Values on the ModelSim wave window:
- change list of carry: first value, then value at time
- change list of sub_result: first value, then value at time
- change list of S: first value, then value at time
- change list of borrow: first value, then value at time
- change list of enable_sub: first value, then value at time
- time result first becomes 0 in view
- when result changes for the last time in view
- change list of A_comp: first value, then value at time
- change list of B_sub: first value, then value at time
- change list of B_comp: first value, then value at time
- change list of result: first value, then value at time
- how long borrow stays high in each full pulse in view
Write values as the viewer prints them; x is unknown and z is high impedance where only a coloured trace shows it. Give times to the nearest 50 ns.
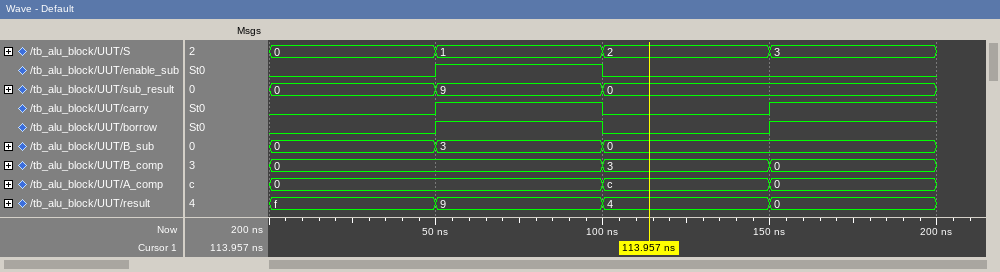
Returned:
0, 1 at 50 ns, 0 at 100 ns, 1 at 150 ns
0, 9 at 50 ns, 0 at 100 ns
0, 1 at 50 ns, 2 at 100 ns, 3 at 150 ns
0, 1 at 50 ns, 0 at 100 ns, 1 at 150 ns
0, 1 at 50 ns, 0 at 100 ns
150 ns
150 ns
0, c at 100 ns, 0 at 150 ns
0, 3 at 50 ns, 0 at 100 ns
0, 3 at 100 ns, 0 at 150 ns
f, 9 at 50 ns, 4 at 100 ns, 0 at 150 ns
50 ns
